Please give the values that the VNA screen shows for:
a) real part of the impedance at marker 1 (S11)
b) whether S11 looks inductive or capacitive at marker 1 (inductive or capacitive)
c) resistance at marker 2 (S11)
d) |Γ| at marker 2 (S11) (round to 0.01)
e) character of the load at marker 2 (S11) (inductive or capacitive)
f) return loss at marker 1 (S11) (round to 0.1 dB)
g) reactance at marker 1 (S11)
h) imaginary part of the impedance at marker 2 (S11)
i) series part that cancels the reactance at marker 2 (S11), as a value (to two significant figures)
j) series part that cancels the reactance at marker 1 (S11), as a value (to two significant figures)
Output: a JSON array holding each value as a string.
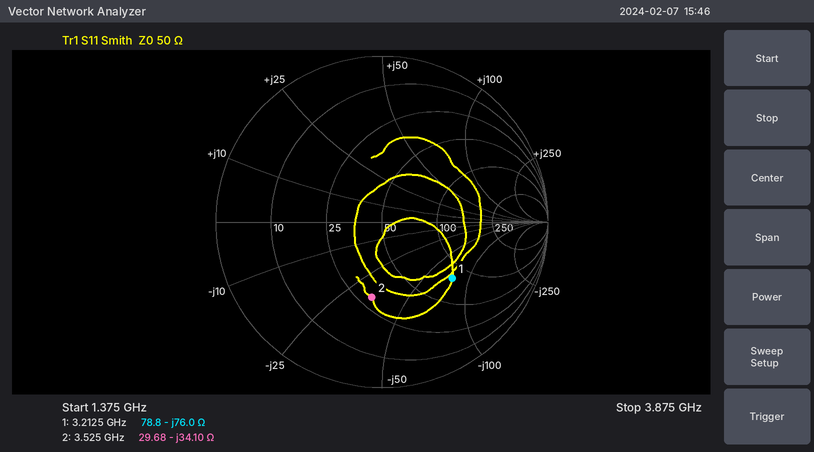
["78.8 Ω", "capacitive", "29.68 Ω", "0.46", "capacitive", "5.3 dB", "-76.0 Ω", "-34.10 Ω", "1.5 nH", "3.8 nH"]
